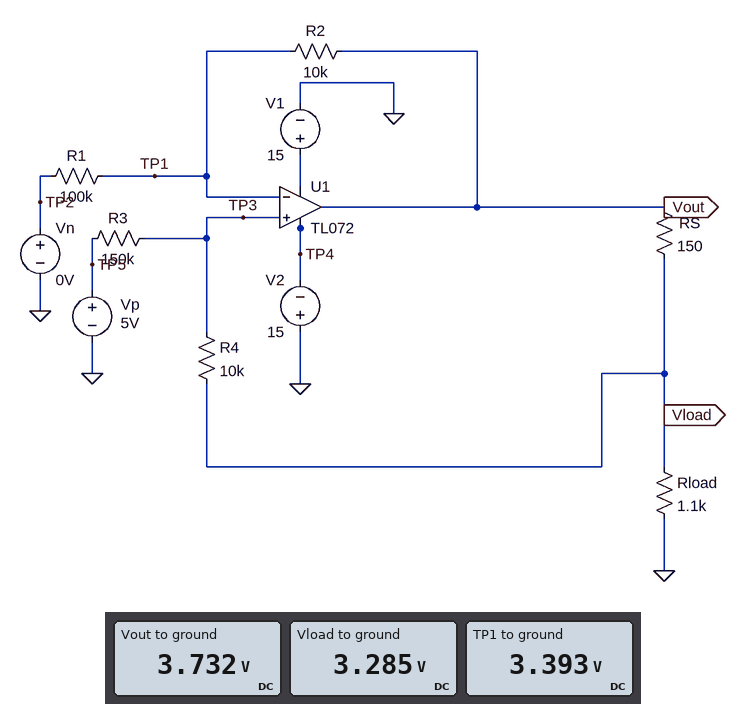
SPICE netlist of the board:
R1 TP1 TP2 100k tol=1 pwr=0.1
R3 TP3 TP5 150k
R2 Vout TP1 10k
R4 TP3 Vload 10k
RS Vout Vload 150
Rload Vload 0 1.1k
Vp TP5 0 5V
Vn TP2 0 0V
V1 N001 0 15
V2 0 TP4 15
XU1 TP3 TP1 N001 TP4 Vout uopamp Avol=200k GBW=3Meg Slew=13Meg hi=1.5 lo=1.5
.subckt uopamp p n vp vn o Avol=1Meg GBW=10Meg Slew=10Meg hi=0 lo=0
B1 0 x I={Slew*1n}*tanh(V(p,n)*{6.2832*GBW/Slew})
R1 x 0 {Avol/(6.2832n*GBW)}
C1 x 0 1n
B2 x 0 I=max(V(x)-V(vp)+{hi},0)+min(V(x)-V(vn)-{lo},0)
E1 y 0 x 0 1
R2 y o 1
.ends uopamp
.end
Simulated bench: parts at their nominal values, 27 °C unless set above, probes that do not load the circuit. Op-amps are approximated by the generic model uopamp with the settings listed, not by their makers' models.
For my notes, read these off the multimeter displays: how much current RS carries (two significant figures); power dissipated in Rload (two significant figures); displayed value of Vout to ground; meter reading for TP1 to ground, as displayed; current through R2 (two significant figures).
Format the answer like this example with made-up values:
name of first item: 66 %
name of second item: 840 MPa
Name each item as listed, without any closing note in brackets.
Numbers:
how much current RS carries: 3.0 mA
power dissipated in Rload: 9.8 mW
displayed value of Vout to ground: 3.732 V
meter reading for TP1 to ground, as displayed: 3.393 V
current through R2: 34 µA
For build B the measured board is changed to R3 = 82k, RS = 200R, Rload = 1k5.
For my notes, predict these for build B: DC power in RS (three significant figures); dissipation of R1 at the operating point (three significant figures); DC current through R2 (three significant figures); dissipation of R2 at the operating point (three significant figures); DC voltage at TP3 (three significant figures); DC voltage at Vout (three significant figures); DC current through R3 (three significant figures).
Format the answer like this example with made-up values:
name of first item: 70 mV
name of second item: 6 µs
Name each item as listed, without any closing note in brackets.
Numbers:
DC power in RS: 1.36 mW
dissipation of R1 at the operating point: 163 µW
DC current through R2: 40.4 µA
dissipation of R2 at the operating point: 16.3 µW
DC voltage at TP3: 4.04 V
DC voltage at Vout: 4.45 V
DC current through R3: 11.7 µA
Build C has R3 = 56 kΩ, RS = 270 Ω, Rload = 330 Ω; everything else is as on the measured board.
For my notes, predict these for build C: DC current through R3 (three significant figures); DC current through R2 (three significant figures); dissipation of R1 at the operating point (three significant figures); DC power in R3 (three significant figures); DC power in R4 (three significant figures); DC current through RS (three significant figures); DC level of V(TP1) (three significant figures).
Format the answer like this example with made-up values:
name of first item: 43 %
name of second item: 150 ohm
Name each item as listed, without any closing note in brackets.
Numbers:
DC current through R3: 61.2 µA
DC current through R2: 15.7 µA
dissipation of R1 at the operating point: 24.7 µW
DC power in R3: 210 µW
DC power in R4: 37.5 µW
DC current through RS: 2.85 mA
DC level of V(TP1): 1.57 V
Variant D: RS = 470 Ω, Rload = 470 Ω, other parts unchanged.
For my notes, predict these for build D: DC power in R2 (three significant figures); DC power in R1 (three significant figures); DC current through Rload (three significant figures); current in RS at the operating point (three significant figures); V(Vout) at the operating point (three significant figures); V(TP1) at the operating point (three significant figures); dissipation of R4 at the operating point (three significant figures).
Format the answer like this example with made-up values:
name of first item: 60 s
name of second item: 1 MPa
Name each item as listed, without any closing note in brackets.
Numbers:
DC power in R2: 433 nW
DC power in R1: 4.33 µW
DC current through Rload: 785 µA
current in RS at the operating point: 756 µA
V(Vout) at the operating point: 724 mV
V(TP1) at the operating point: 658 mV
dissipation of R4 at the operating point: 8.38 µW
